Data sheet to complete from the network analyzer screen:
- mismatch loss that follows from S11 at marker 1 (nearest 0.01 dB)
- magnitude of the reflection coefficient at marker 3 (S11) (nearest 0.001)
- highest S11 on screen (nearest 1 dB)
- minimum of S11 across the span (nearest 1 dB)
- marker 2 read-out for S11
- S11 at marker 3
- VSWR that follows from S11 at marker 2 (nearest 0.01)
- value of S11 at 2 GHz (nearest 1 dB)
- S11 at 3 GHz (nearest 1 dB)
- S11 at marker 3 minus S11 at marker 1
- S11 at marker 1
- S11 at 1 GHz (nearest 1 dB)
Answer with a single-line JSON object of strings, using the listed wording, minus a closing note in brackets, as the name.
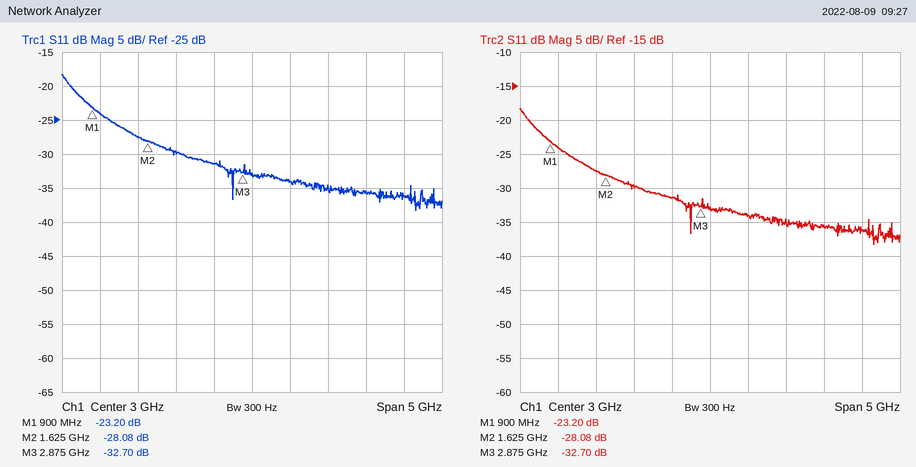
{"mismatch loss that follows from S11 at marker 1": "0.02 dB", "magnitude of the reflection coefficient at marker 3 (S11)": "0.023", "highest S11 on screen": "-18 dB", "minimum of S11 across the span": "-38 dB", "marker 2 read-out for S11": "-28.08 dB", "S11 at marker 3": "-32.70 dB", "VSWR that follows from S11 at marker 2": "1.08", "value of S11 at 2 GHz": "-30 dB", "S11 at 3 GHz": "-33 dB", "S11 at marker 3 minus S11 at marker 1": "-9.50 dB", "S11 at marker 1": "-23.20 dB", "S11 at 1 GHz": "-24 dB"}
